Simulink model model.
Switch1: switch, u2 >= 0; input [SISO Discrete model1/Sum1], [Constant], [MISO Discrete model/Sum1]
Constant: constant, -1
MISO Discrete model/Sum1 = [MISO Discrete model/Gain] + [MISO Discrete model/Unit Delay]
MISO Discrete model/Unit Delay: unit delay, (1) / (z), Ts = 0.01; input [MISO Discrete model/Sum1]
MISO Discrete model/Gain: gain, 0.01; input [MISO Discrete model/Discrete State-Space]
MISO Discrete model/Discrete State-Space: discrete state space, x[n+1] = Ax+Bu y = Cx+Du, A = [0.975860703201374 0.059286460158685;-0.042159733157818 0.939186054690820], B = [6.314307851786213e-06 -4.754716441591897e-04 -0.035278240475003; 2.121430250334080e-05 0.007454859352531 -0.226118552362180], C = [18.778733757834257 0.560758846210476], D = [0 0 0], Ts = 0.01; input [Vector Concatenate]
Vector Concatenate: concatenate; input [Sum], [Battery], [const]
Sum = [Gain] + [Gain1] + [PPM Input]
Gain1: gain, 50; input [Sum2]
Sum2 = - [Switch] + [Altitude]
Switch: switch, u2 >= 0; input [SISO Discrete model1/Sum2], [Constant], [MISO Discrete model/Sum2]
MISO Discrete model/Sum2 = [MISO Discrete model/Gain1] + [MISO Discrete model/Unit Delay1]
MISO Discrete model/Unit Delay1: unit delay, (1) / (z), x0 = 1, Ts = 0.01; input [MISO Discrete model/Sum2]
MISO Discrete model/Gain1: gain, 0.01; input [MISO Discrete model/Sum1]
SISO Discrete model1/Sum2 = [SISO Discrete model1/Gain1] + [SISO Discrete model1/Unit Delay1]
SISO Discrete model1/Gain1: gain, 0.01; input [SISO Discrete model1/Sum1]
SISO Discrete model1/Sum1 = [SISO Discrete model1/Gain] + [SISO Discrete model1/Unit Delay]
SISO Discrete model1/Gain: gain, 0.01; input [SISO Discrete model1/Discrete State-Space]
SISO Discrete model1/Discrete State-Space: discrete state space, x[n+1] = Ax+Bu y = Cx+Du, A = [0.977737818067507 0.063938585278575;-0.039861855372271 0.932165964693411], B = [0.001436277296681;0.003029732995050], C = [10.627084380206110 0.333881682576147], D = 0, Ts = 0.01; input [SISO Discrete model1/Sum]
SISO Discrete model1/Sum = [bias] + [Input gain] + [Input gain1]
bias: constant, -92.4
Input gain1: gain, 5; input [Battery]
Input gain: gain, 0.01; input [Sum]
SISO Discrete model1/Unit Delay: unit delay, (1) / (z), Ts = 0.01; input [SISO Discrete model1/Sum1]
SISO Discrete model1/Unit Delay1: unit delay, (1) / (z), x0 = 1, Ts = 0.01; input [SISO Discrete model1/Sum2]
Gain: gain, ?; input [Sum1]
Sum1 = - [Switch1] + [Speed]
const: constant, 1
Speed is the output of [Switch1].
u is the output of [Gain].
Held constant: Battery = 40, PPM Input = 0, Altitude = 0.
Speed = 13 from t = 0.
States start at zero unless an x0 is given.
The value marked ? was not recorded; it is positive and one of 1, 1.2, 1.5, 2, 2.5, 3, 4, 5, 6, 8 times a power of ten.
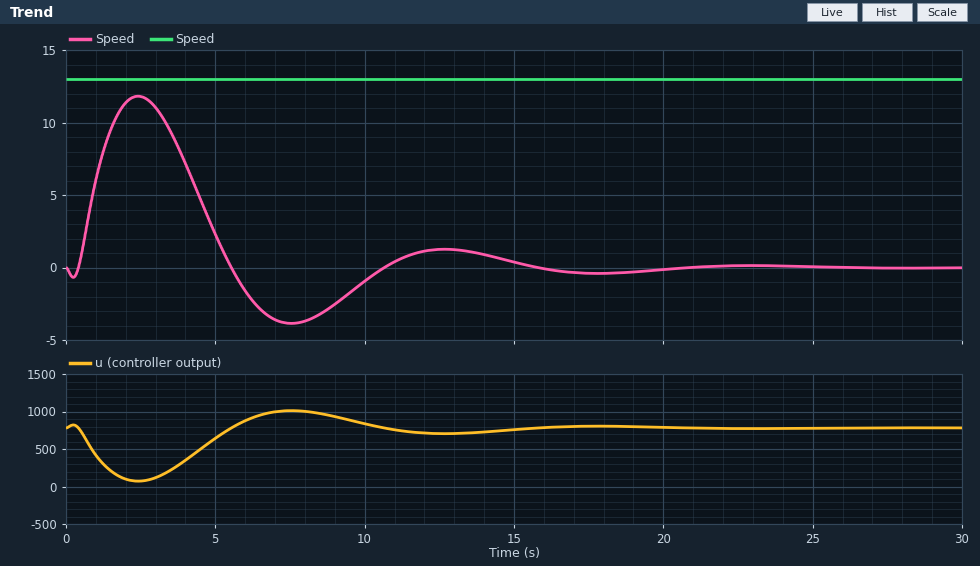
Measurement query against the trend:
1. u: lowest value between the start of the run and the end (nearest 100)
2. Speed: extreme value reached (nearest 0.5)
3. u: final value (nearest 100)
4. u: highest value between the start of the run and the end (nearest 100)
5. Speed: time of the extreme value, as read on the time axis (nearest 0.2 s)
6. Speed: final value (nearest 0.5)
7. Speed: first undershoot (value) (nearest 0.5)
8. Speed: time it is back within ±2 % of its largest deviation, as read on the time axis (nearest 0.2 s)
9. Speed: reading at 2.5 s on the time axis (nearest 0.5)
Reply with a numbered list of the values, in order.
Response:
1. 100
2. 12.0
3. 800
4. 1000
5. 2.4 s
6. 0.0
7. -4.0
8. 19.4 s
9. 12.0
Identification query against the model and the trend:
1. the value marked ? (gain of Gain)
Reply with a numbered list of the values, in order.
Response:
1. 60
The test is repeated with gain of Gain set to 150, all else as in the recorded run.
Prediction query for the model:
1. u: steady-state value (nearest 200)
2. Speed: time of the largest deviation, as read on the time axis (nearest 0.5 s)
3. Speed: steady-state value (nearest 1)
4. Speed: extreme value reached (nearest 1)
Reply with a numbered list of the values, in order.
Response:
1. 2000
2. 1.5 s
3. 0
4. 13
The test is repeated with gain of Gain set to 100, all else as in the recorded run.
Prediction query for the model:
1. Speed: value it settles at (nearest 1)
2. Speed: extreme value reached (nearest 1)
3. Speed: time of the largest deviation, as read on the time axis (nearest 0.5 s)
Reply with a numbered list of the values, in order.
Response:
1. 0
2. 13
3. 2.0 s
